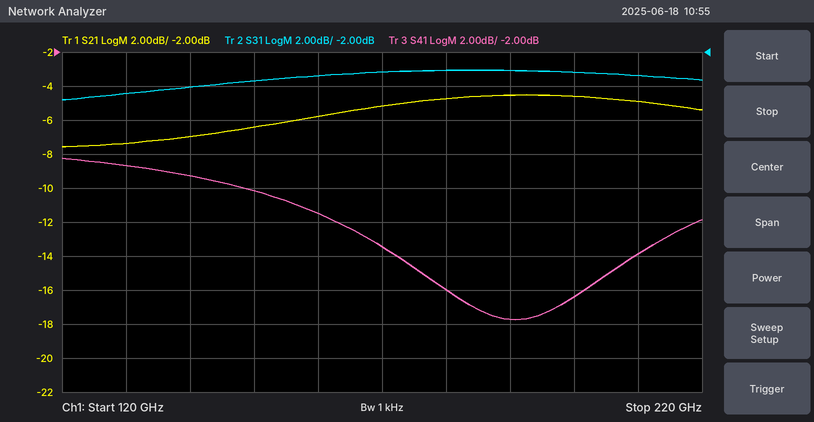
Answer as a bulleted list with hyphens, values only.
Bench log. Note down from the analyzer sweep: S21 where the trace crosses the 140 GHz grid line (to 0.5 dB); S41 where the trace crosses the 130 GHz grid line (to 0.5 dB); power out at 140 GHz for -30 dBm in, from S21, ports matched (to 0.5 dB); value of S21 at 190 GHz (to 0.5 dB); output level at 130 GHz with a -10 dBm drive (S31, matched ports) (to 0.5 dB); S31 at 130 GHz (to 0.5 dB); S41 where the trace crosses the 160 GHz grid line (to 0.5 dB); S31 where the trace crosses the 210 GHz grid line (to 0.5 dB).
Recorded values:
- -7.0 dB
- -8.5 dB
- -37.0 dBm
- -4.5 dB
- -14.5 dBm
- -4.5 dB
- -11.5 dB
- -3.5 dB
